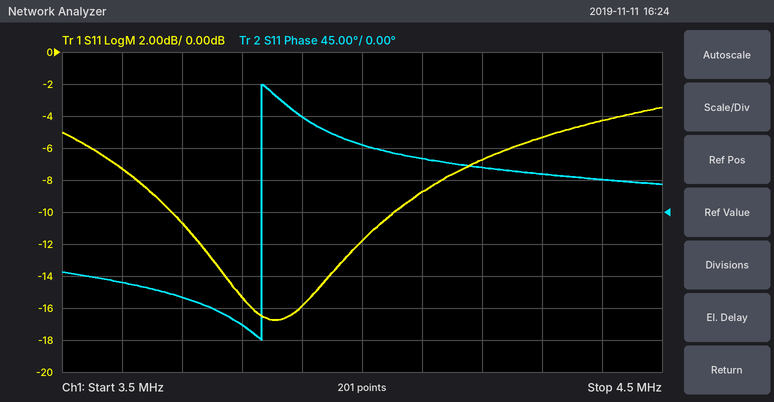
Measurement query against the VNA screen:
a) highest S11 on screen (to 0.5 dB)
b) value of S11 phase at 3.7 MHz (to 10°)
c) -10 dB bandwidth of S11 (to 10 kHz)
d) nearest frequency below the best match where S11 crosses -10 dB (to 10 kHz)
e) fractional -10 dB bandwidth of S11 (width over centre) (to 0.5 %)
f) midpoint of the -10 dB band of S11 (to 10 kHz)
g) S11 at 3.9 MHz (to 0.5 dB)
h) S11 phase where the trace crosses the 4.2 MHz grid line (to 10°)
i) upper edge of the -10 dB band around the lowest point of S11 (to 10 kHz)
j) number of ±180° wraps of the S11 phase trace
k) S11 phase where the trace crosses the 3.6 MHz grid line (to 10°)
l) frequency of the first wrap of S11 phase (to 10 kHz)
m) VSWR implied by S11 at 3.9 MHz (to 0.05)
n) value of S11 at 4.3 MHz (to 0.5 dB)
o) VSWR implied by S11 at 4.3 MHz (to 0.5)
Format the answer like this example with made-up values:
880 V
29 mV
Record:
-3.5 dB
-120°
370 kHz
3.68 MHz
9.5 %
3.87 MHz
-16.0 dB
60°
4.05 MHz
1
-100°
3.83 MHz
1.40
-5.5 dB
3.5
